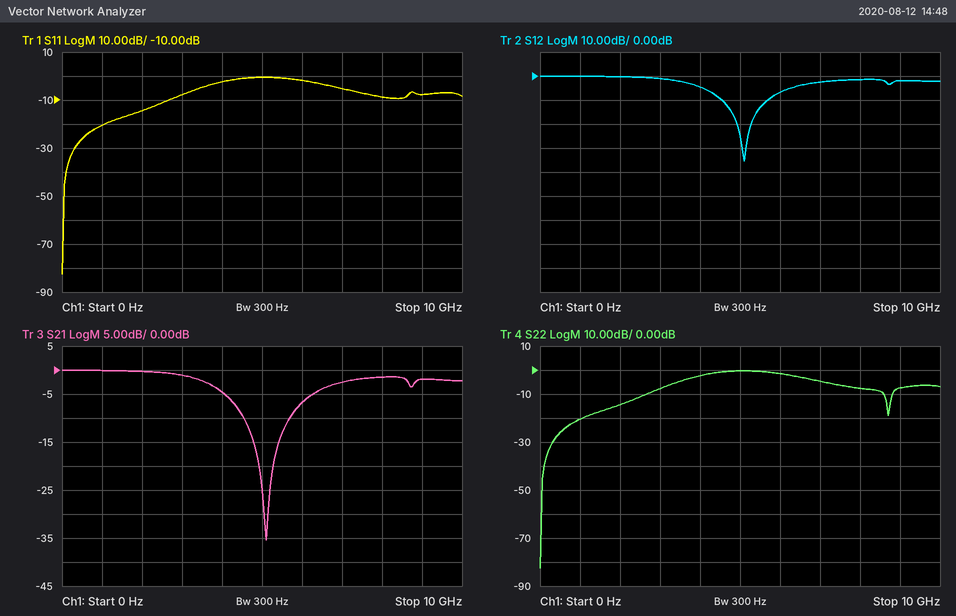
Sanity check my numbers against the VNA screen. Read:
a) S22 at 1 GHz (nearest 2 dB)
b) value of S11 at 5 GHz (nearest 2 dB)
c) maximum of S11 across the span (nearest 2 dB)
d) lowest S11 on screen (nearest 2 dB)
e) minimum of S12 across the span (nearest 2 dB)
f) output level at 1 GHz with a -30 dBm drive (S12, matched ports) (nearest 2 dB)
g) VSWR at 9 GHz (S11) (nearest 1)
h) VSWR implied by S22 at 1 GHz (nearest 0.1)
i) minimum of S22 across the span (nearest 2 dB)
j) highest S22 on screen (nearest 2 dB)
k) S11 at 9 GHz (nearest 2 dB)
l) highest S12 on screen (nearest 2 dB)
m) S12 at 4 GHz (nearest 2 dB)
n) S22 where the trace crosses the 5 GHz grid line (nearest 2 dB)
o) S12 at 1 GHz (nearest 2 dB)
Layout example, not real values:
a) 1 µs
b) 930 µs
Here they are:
a) -20 dB
b) 0 dB
c) 0 dB
d) -82 dB
e) -36 dB
f) -30 dBm
g) 2
h) 1.2
i) -82 dB
j) 0 dB
k) -8 dB
l) 0 dB
m) -4 dB
n) 0 dB
o) 0 dB
